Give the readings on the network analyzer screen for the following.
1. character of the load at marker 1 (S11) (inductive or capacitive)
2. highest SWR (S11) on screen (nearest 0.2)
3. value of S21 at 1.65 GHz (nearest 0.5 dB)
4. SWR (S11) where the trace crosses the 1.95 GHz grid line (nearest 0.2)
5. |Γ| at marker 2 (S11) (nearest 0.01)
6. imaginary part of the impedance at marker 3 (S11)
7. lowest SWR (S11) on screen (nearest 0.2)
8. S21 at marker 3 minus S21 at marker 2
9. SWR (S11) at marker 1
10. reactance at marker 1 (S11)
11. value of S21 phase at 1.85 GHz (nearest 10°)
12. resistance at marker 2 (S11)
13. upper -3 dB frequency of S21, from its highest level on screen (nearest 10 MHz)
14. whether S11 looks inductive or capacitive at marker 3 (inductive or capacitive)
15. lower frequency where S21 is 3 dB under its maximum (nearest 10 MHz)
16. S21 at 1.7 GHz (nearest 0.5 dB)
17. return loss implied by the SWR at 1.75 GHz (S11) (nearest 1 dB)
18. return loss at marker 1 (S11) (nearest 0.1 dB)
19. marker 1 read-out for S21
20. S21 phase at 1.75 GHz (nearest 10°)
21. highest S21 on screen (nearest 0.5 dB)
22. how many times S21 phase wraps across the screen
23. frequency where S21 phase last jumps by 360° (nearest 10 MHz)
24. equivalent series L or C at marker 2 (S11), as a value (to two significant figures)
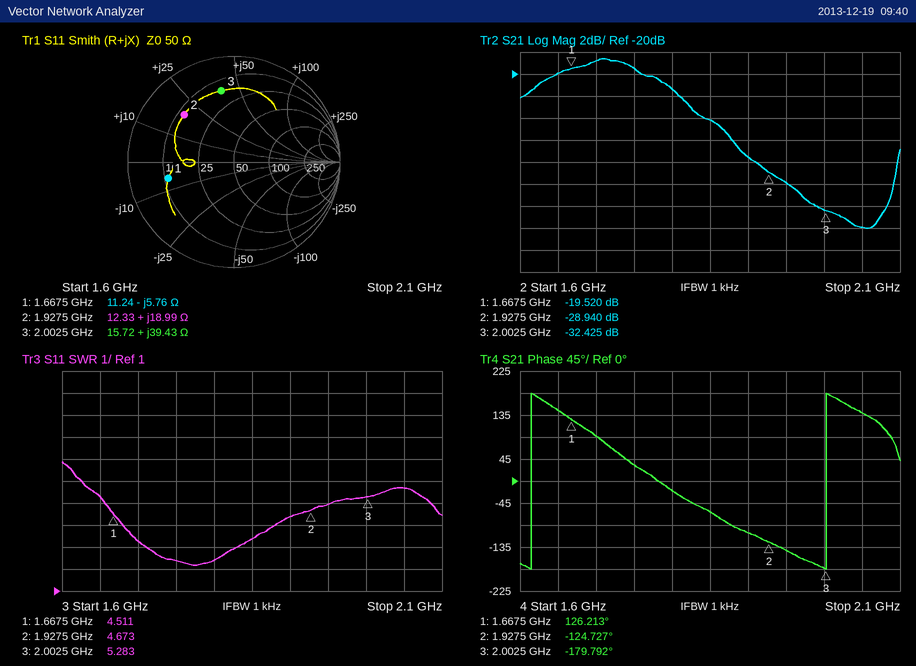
capacitive
6.8
-20.0 dB
5.0
0.65
+39.43 Ω
2.2
-3.485 dB
4.511
-5.76 Ω
-60°
12.33 Ω
1.80 GHz
inductive
1.61 GHz
-19.0 dB
8 dB
3.9 dB
-19.520 dB
30°
-18.5 dB
2
2.00 GHz
1.6 nH
